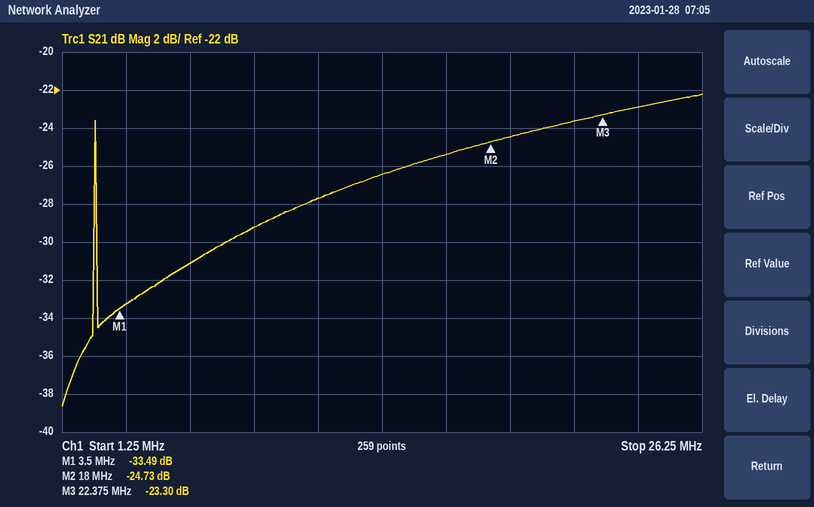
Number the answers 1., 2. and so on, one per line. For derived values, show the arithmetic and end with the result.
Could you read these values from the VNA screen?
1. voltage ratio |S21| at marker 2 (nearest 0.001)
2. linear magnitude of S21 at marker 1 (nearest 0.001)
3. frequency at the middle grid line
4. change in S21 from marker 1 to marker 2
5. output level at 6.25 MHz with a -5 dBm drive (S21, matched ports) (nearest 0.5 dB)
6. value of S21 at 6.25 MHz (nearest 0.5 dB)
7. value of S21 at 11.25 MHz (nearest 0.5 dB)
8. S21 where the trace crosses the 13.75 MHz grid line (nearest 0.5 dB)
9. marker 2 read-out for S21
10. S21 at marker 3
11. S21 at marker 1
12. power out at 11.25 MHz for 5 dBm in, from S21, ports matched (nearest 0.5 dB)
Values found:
1. 10^(-24.73/20) ≈ 0.058
2. 10^(-33.49/20) ≈ 0.021
3. 13.75 MHz
4. -24.73 − (-33.49) = 8.76 dB
5. -5 dBm + (-31.0 dB) = -36.0 dBm
6. -31.0 dB
7. -27.5 dB
8. -26.5 dB
9. -24.73 dB
10. -23.30 dB
11. -33.49 dB
12. 5 dBm + (-27.5 dB) = -22.5 dBm
